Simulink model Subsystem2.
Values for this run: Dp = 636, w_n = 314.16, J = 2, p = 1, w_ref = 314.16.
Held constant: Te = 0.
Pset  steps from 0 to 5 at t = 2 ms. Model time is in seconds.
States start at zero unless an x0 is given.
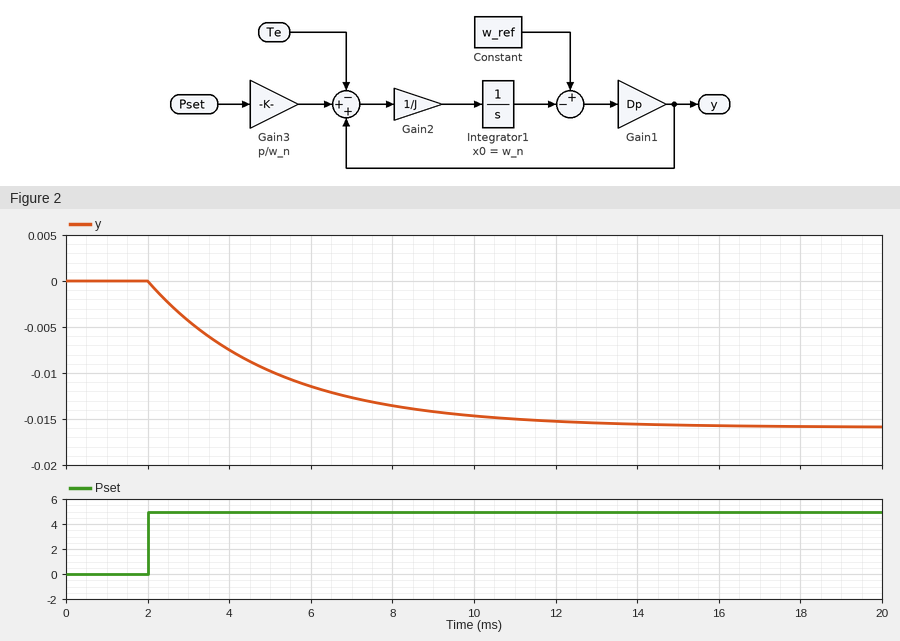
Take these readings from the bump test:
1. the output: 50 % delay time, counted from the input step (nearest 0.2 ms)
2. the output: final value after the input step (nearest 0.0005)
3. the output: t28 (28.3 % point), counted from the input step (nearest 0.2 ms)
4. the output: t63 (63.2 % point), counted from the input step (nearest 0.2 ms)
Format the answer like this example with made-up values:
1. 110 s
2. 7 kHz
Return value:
1. 2.2 ms
2. -0.0160
3. 1.0 ms
4. 3.2 ms
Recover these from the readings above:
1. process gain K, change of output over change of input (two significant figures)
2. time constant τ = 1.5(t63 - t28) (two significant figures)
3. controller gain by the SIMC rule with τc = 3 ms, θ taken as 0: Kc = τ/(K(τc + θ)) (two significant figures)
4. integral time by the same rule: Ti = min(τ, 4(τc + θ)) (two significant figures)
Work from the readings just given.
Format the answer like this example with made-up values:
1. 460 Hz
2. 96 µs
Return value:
1. -0.0032
2. 3.3 ms
3. -340
4. 3.3 ms
